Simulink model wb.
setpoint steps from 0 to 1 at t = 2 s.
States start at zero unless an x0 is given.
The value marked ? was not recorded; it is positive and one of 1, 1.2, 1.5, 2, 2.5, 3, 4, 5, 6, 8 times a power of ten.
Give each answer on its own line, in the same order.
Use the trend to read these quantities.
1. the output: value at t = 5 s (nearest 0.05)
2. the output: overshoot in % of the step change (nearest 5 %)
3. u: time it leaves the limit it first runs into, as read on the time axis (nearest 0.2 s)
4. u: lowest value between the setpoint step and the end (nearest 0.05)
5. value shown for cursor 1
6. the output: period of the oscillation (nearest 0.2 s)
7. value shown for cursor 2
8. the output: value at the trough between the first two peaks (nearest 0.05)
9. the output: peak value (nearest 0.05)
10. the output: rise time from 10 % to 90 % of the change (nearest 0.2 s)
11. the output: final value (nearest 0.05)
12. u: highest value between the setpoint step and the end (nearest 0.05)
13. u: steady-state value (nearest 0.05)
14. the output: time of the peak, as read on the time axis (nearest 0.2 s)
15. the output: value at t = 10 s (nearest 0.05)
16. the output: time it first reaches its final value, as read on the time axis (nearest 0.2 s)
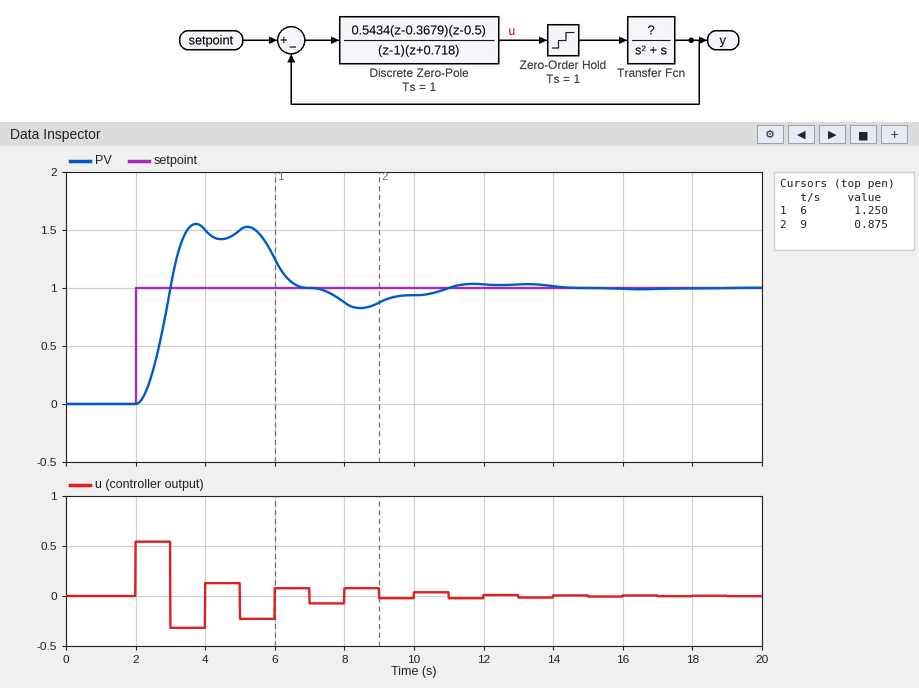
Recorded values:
1.50
55 %
3.0 s
-0.30
1.250
1.4 s
0.875
1.40
1.55
0.6 s
1.00
0.55
0.00
3.8 s
0.95
3.0 s
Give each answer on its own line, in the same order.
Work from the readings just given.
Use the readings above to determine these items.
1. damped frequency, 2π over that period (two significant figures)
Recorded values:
4.5 rad/s
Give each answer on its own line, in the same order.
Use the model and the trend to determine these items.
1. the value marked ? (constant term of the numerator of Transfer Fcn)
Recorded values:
5
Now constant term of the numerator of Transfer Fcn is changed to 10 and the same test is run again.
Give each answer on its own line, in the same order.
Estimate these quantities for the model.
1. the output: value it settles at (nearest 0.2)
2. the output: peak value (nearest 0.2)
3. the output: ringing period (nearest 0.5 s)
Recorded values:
1.0
2.6
2.0 s
